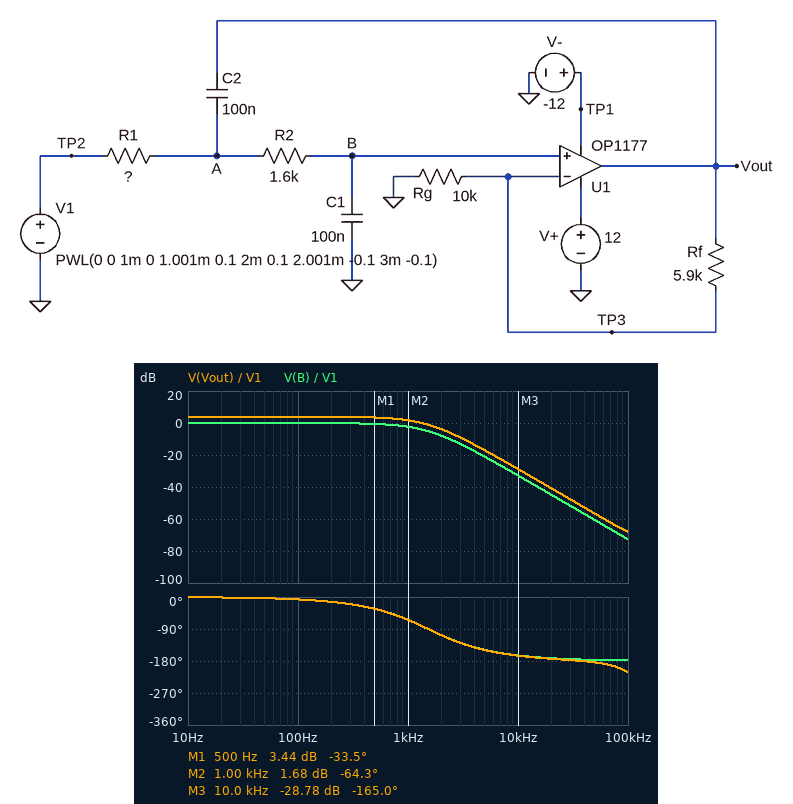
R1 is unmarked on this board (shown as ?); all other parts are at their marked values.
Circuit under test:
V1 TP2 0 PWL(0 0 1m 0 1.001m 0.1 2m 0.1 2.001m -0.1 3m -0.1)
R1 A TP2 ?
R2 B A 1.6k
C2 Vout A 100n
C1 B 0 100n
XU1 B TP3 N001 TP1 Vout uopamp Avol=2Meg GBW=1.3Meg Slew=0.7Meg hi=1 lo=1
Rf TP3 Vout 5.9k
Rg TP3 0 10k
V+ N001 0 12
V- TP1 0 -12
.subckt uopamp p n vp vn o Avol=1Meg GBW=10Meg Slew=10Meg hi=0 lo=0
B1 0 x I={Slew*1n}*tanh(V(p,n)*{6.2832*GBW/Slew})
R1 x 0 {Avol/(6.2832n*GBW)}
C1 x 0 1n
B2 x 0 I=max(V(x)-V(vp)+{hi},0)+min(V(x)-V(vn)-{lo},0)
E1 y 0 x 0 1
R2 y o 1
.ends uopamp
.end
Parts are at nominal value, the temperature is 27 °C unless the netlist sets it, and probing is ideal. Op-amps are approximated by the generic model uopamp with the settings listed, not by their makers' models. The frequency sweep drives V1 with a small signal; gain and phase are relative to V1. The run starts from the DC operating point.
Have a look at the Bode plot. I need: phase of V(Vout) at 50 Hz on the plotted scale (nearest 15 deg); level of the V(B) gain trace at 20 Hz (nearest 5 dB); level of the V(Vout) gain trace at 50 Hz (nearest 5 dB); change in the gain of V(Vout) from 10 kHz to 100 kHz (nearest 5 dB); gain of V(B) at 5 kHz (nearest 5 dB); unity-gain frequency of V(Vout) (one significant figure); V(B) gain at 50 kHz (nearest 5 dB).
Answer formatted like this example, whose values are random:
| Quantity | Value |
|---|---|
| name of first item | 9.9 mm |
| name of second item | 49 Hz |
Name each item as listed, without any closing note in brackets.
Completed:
| Quantity | Value |
|---|---|
| phase of V(Vout) at 50 Hz on the plotted scale | 0 deg |
| level of the V(B) gain trace at 20 Hz | 0 dB |
| level of the V(Vout) gain trace at 50 Hz | 5 dB |
| change in the gain of V(Vout) from 10 kHz to 100 kHz | -40 dB |
| gain of V(B) at 5 kHz | -20 dB |
| unity-gain frequency of V(Vout) | 1 kHz |
| V(B) gain at 50 kHz | -60 dB |
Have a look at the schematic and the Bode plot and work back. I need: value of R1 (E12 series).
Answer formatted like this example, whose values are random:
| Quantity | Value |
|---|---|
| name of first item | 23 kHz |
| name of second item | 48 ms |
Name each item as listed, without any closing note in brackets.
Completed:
| Quantity | Value |
|---|---|
| value of R1 | 680 Ω |
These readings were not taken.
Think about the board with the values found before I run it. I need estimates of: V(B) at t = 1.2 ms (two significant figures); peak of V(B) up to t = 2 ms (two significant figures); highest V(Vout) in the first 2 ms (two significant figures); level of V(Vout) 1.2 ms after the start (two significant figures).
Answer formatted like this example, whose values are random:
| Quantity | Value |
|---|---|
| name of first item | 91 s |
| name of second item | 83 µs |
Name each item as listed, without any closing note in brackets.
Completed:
| Quantity | Value |
|---|---|
| V(B) at t = 1.2 ms | 61 mV |
| peak of V(B) up to t = 2 ms | 100 mV |
| highest V(Vout) in the first 2 ms | 160 mV |
| level of V(Vout) 1.2 ms after the start | 96 mV |
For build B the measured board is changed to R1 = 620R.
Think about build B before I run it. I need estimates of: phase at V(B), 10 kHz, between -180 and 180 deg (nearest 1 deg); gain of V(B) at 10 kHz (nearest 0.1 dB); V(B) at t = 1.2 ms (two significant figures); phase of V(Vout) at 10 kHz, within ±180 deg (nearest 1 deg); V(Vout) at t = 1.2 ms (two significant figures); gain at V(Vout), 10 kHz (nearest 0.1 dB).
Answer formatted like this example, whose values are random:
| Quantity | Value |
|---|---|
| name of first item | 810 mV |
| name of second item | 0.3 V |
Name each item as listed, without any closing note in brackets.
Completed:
| Quantity | Value |
|---|---|
| phase at V(B), 10 kHz, between -180 and 180 deg | -163 deg |
| gain of V(B) at 10 kHz | -32.0 dB |
| V(B) at t = 1.2 ms | 62 mV |
| phase of V(Vout) at 10 kHz, within ±180 deg | -164 deg |
| V(Vout) at t = 1.2 ms | 99 mV |
| gain at V(Vout), 10 kHz | -28.0 dB |
